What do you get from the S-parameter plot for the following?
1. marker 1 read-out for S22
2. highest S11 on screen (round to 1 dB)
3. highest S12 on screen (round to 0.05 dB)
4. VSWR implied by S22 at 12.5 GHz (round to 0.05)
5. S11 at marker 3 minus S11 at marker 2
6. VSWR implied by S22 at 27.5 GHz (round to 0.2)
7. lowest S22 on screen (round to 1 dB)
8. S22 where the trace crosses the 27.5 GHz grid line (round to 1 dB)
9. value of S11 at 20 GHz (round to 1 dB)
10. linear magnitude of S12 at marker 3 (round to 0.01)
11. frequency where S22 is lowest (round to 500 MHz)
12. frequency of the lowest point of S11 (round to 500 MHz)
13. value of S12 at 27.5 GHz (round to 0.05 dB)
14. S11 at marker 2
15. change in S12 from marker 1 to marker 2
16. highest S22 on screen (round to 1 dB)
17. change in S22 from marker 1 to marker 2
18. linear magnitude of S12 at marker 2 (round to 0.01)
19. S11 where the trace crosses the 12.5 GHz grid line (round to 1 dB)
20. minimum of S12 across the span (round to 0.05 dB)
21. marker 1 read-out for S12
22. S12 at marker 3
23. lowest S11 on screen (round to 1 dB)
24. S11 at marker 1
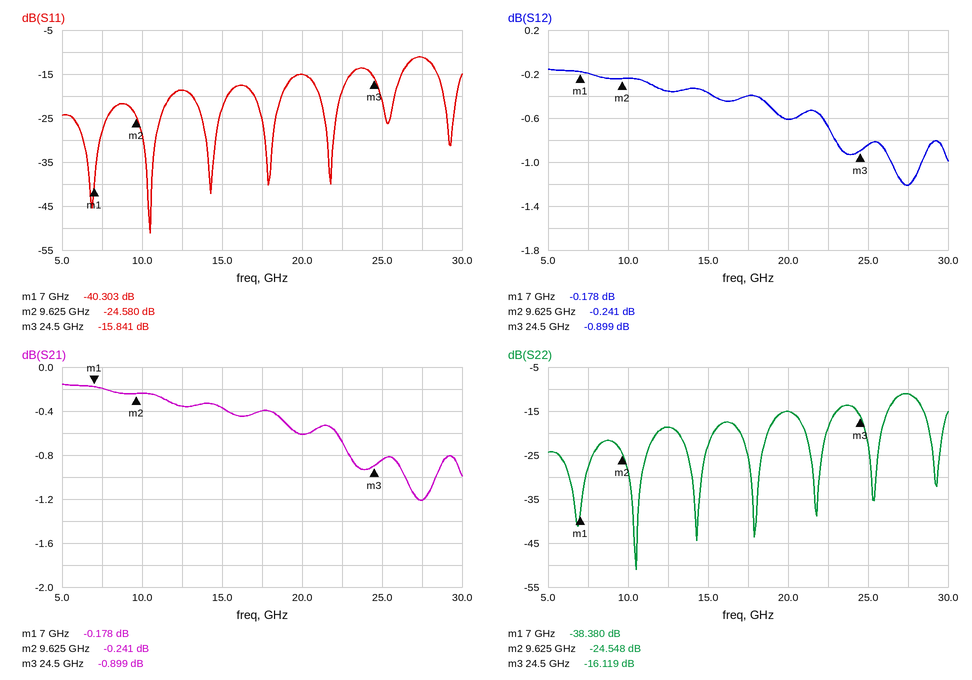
-38.380 dB
-11 dB
-0.15 dB
1.25
8.739 dB
1.8
-51 dB
-11 dB
-15 dB
0.90
10.5 GHz
10.5 GHz
-1.20 dB
-24.580 dB
-0.063 dB
-11 dB
13.832 dB
0.97
-19 dB
-1.20 dB
-0.178 dB
-0.899 dB
-51 dB
-40.303 dB
